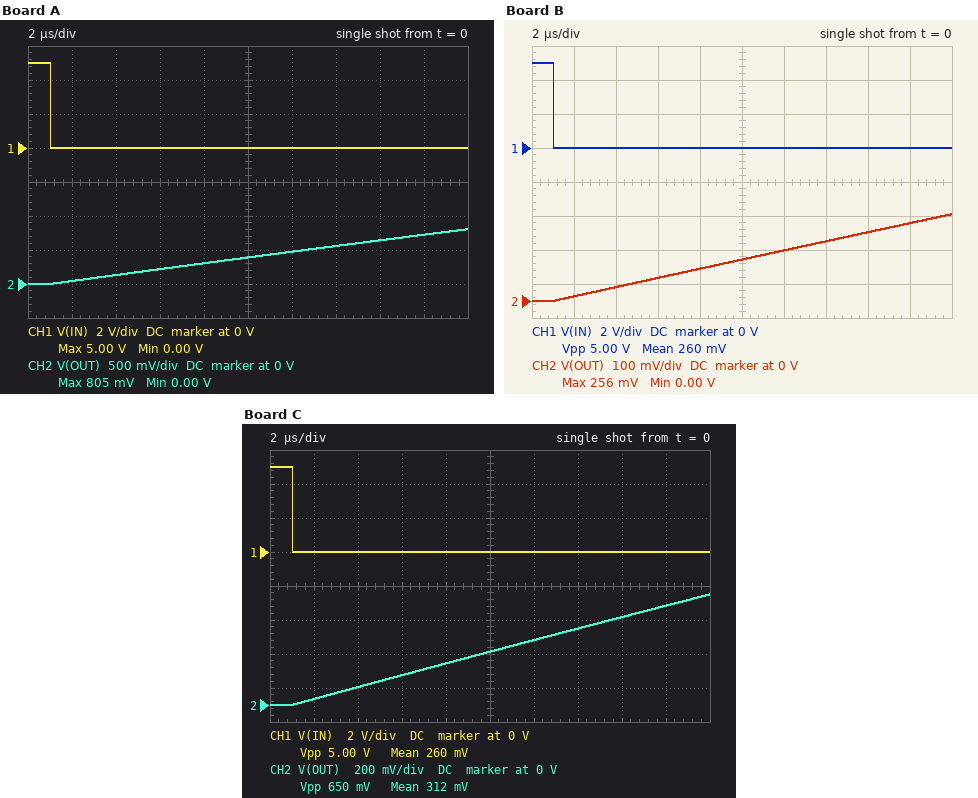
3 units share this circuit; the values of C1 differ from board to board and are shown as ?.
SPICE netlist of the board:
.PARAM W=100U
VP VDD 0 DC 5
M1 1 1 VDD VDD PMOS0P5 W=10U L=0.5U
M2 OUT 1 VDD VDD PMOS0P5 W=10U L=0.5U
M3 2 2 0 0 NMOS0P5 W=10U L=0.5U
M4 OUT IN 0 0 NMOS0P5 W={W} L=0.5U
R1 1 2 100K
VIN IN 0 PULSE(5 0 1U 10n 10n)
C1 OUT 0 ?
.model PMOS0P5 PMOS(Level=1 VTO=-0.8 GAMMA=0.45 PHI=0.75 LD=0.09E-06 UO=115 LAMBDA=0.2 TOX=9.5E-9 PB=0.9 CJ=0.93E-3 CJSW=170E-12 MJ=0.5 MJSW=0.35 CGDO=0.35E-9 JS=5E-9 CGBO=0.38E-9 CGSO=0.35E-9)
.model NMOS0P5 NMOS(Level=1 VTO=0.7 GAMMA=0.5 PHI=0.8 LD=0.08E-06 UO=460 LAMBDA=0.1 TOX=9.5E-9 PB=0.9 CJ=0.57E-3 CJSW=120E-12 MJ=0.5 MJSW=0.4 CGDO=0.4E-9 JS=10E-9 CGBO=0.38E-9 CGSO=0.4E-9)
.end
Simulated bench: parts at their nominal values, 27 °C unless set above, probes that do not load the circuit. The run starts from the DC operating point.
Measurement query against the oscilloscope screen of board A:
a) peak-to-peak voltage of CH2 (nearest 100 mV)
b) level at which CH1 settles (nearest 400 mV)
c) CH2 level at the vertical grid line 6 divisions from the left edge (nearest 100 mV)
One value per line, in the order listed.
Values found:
800 mV
0 V
500 mV
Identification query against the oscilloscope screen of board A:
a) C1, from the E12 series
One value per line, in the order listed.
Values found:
1.2 nF
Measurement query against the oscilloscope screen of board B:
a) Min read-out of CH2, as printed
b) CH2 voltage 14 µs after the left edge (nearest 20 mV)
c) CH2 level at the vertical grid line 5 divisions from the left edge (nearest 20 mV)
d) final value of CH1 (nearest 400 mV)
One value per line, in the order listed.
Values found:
0.00 V
180 mV
120 mV
0 V
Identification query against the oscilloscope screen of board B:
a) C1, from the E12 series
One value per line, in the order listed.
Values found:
3.9 nF
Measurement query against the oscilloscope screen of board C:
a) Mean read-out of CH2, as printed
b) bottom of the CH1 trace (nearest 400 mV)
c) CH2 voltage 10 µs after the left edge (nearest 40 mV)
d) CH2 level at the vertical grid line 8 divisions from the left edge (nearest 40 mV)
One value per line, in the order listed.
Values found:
312 mV
0 V
320 mV
520 mV
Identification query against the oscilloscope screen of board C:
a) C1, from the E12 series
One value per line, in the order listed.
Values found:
1.5 nF
